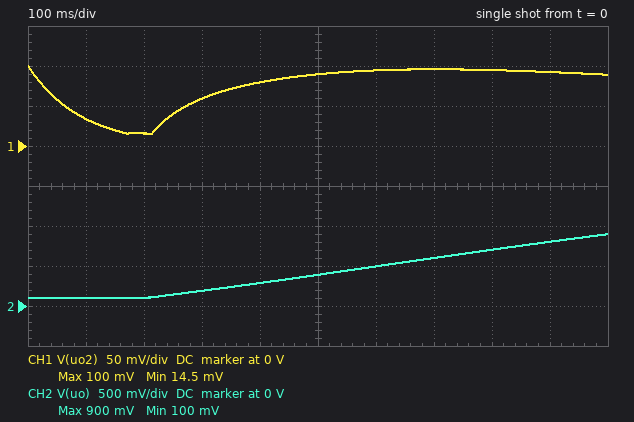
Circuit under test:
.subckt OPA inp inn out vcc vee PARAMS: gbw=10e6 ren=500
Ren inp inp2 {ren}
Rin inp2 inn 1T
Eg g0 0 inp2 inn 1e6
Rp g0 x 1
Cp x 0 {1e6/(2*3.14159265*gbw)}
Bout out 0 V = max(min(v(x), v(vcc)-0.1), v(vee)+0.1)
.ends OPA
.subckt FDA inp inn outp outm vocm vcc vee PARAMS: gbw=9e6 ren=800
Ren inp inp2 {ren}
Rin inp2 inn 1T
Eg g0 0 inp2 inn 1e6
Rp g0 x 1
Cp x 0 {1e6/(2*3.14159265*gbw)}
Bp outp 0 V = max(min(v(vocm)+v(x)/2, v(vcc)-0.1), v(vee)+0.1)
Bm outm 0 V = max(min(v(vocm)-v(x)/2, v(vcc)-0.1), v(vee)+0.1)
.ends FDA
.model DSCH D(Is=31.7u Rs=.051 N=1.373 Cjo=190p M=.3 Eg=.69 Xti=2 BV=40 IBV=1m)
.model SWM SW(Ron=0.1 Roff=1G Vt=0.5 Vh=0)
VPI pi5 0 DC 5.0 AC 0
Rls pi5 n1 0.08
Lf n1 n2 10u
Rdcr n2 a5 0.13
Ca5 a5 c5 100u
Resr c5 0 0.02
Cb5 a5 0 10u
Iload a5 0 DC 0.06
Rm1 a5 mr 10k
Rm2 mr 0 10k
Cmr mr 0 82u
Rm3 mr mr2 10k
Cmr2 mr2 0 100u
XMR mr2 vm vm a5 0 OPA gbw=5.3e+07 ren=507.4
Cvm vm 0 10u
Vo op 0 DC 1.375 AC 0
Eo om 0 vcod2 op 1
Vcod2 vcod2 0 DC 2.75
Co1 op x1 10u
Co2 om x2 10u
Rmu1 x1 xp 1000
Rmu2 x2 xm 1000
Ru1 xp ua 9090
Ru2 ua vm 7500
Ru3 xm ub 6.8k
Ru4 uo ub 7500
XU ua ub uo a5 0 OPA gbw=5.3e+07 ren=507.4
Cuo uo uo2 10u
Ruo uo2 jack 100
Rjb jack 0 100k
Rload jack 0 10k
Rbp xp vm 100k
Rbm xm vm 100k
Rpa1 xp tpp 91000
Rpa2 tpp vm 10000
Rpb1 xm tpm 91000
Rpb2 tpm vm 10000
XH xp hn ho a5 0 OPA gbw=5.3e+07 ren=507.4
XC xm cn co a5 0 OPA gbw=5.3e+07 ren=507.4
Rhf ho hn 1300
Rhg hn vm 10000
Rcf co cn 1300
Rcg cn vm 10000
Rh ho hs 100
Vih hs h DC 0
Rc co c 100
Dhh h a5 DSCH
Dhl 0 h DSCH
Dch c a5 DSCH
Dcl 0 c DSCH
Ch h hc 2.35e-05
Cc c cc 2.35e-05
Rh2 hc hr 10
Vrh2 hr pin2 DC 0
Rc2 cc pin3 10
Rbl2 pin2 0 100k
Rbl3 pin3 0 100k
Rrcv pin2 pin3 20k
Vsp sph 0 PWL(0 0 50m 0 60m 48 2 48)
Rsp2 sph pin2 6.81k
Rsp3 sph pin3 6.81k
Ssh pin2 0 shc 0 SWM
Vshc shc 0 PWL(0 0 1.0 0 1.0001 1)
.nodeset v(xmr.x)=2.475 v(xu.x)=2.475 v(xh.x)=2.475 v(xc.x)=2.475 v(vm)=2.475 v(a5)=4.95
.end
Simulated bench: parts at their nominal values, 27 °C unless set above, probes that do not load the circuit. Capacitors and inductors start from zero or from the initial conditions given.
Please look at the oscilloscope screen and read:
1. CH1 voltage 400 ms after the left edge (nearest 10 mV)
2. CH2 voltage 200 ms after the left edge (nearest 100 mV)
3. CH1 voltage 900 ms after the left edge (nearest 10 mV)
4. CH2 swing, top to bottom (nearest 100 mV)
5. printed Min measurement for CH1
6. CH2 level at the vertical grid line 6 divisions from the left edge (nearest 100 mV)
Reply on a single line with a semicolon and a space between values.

80 mV; 100 mV; 90 mV; 800 mV; 14.5 mV; 500 mV
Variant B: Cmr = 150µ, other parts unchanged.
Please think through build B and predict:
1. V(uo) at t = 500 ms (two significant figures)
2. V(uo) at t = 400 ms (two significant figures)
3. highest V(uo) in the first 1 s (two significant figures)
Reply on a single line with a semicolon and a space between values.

270 mV; 190 mV; 700 mV
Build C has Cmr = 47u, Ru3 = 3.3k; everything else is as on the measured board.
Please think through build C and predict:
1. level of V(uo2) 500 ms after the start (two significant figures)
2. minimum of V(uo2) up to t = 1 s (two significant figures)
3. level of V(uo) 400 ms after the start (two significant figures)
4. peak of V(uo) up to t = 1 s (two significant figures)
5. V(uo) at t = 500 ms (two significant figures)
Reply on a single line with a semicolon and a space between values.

100 mV; 19 mV; 400 mV; 1.0 V; 510 mV
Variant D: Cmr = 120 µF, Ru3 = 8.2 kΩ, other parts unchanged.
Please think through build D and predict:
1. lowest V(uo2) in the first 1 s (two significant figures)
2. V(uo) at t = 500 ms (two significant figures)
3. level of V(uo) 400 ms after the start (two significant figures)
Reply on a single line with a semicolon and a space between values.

7.8 mV; 310 mV; 220 mV
